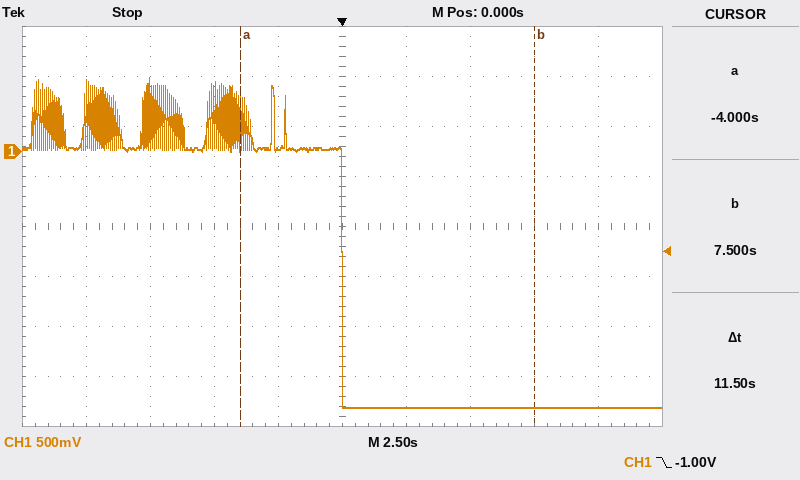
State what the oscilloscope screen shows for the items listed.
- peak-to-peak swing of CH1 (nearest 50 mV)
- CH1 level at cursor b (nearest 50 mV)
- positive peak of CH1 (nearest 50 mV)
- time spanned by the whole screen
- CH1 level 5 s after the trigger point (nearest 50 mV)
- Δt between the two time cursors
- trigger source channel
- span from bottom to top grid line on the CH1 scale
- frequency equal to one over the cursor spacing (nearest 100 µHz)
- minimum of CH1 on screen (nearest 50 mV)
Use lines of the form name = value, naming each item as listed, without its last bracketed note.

peak-to-peak swing of CH1 = 3.30 V
CH1 level at cursor b = -2.55 V
positive peak of CH1 = 750 mV
time spanned by the whole screen = 25 s
CH1 level 5 s after the trigger point = -2.55 V
Δt between the two time cursors = 11.5 s
trigger source channel = CH1
span from bottom to top grid line on the CH1 scale = 4 V
frequency equal to one over the cursor spacing = 87.0 mHz
minimum of CH1 on screen = -2.55 V
